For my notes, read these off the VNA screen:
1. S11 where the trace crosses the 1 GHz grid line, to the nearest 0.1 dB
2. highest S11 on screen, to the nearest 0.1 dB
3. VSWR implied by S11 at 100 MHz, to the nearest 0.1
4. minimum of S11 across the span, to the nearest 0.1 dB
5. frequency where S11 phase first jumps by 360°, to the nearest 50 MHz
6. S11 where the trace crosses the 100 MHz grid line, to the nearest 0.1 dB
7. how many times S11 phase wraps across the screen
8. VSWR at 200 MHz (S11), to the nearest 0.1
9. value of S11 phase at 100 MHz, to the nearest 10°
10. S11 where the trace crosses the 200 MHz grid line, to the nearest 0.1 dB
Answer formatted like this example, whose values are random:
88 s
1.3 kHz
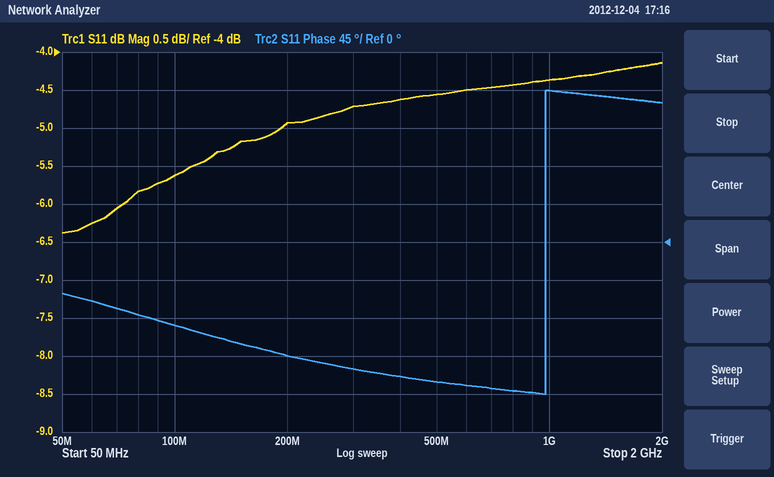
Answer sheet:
-4.4 dB
-4.1 dB
3.2
-6.4 dB
1.00 GHz
-5.6 dB
1
3.6
-100°
-4.9 dB
